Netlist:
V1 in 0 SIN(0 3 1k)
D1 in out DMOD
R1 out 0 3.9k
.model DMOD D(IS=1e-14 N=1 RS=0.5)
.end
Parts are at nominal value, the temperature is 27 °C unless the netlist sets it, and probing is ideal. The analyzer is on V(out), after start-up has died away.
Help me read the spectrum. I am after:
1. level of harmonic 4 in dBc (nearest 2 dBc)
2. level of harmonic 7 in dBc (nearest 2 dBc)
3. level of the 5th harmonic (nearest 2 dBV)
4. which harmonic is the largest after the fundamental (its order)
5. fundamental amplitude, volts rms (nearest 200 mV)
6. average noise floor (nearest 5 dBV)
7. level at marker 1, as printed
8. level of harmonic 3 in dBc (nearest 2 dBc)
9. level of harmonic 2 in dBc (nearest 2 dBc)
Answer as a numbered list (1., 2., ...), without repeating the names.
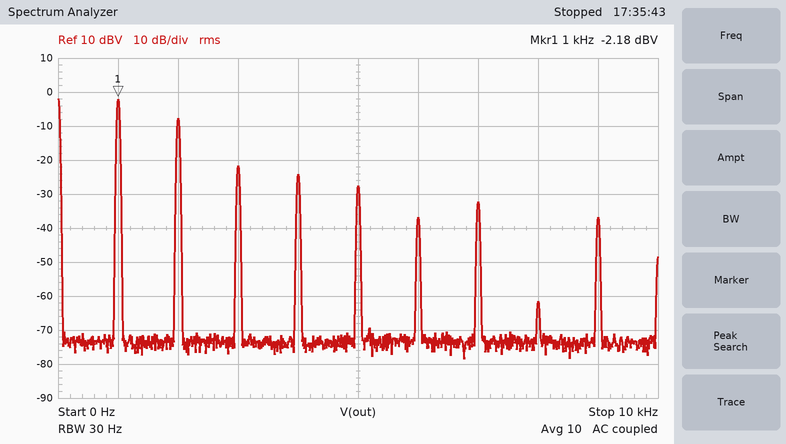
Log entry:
1. -22 dBc
2. -30 dBc
3. -28 dBV
4. 2
5. 800 mV
6. -75 dBV
7. -2.18 dBV
8. -20 dBc
9. -6 dBc
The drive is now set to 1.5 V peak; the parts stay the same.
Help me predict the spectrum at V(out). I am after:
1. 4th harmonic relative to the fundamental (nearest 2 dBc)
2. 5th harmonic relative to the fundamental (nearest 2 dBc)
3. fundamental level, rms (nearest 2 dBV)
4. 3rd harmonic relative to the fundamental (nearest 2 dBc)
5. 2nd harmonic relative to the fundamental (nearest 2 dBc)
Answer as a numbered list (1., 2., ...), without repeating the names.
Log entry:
1. -36 dBc
2. -22 dBc
3. -12 dBV
4. -12 dBc
5. -4 dBc
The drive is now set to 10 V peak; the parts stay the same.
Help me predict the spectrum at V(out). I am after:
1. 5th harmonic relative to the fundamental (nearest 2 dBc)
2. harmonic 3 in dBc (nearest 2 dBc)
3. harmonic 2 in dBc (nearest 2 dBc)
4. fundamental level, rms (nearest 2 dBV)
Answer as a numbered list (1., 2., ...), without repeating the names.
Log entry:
1. -36 dBc
2. -30 dBc
3. -6 dBc
4. 10 dBV
